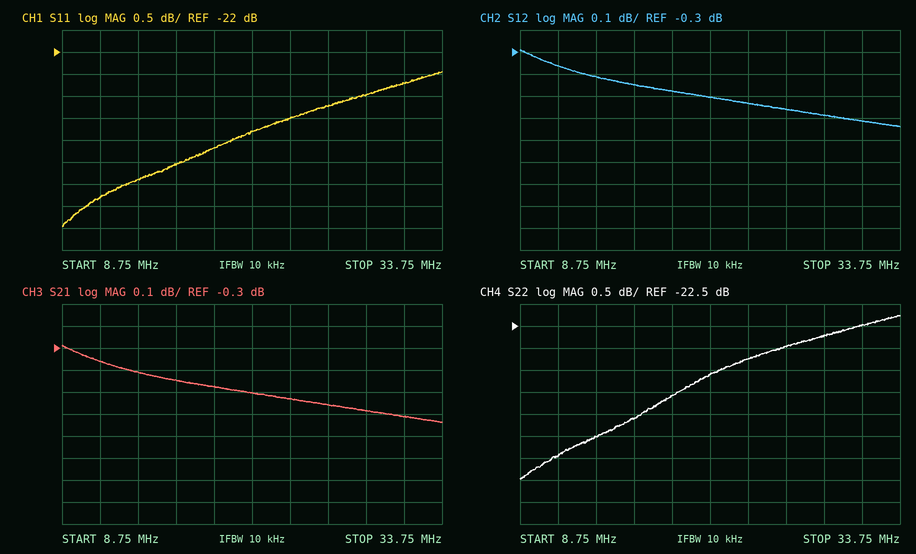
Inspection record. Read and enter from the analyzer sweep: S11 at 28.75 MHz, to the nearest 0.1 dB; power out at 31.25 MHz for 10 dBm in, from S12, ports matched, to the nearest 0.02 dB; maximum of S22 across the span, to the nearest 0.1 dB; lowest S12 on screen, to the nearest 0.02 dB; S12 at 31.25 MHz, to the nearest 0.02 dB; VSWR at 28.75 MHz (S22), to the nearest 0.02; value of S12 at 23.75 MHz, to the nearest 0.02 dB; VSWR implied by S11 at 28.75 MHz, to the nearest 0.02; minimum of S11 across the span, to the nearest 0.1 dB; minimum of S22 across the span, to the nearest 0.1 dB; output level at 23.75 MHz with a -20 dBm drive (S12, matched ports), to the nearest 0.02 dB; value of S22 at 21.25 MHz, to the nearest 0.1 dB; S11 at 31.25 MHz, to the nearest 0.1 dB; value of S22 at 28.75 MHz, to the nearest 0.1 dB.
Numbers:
-23.0 dB
9.38 dBm
-22.3 dB
-0.64 dB
-0.62 dB
1.16
-0.54 dB
1.16
-26.0 dB
-26.0 dB
-20.54 dBm
-23.6 dB
-22.7 dB
-22.7 dB
